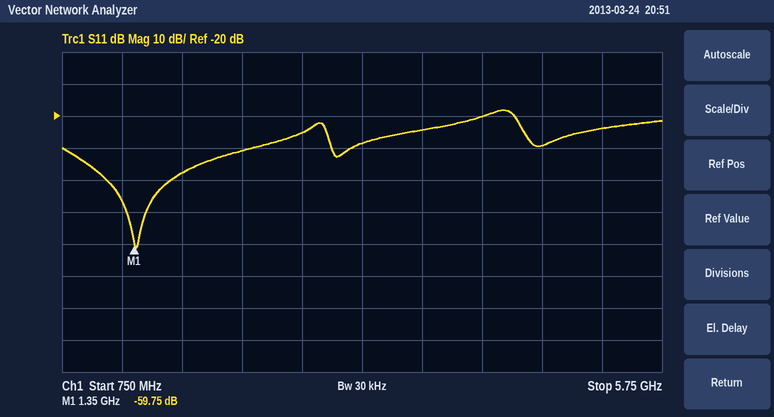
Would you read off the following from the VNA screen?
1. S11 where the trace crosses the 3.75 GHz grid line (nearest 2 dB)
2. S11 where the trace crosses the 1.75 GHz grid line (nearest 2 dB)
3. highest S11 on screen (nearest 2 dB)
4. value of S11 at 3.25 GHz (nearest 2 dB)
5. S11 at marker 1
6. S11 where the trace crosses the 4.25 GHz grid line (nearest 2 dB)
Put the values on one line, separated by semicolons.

-24 dB; -38 dB; -18 dB; -28 dB; -59.75 dB; -20 dB
